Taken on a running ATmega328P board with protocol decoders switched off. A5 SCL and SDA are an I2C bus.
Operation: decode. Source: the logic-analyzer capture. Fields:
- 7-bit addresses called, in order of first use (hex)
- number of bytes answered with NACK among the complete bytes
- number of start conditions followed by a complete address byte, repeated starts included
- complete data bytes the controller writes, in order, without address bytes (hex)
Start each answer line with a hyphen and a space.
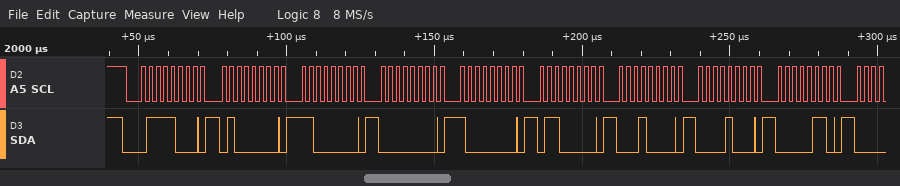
- 0x3C
- 0
- 1
- 40 C0 00 80 60 10 08 06
